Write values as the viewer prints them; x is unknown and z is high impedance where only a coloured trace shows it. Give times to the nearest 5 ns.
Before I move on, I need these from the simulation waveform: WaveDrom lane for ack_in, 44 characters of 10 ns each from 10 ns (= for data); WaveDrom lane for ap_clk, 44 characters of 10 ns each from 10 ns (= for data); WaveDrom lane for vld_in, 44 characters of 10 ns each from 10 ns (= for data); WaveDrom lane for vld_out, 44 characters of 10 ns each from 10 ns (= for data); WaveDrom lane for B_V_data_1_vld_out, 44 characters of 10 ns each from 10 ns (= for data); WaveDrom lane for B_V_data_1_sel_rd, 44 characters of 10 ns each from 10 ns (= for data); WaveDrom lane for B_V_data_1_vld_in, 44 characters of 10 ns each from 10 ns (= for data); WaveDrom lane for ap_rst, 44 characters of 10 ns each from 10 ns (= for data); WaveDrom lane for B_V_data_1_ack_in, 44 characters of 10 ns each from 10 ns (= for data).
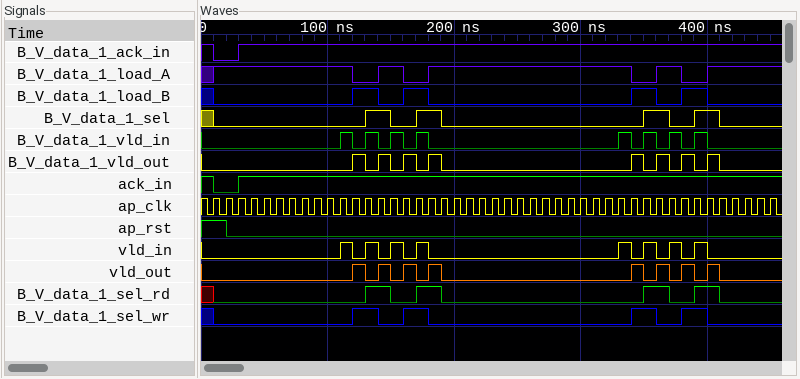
{name: 'ack_in', wave: '0.1.........................................'}
{name: 'ap_clk', wave: 'p...........................................'}
{name: 'vld_in', wave: '0.........10101010..............10101010....'}
{name: 'vld_out', wave: '0..........10101010..............10101010...'}
{name: 'B_V_data_1_vld_out', wave: '0..........10101010..............10101010...'}
{name: 'B_V_data_1_sel_rd', wave: '0...........1.0.1.0...............1.0.1.0...'}
{name: 'B_V_data_1_vld_in', wave: '0.........10101010..............10101010....'}
{name: 'ap_rst', wave: '10..........................................'}
{name: 'B_V_data_1_ack_in', wave: '0.1.........................................'}
